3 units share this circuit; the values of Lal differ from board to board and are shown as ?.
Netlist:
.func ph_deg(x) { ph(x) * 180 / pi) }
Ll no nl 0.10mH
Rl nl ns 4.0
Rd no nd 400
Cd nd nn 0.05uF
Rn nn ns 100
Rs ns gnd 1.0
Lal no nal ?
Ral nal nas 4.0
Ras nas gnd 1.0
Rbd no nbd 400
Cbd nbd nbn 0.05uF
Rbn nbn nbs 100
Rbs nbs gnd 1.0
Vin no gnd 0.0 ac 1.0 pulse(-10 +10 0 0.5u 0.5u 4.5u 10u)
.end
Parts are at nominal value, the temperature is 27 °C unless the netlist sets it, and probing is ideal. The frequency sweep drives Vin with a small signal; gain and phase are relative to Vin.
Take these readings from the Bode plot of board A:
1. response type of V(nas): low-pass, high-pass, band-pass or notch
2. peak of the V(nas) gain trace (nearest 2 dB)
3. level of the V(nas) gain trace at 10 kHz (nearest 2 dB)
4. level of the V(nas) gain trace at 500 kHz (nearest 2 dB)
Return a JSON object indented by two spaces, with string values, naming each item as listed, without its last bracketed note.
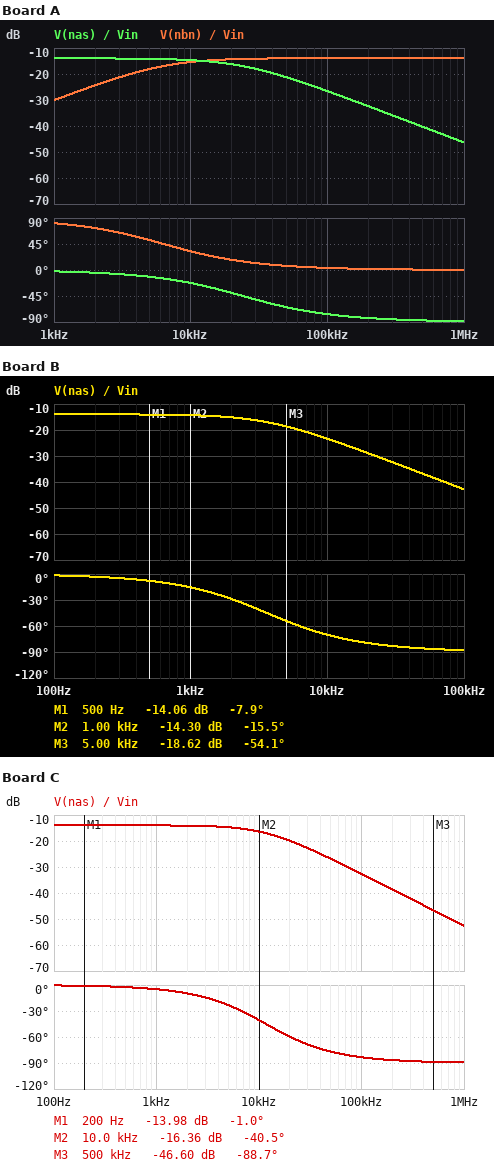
{
  "response type of V(nas): low-pass, high-pass, band-pass or notch": "low-pass",
  "peak of the V(nas) gain trace": "-14 dB",
  "level of the V(nas) gain trace at 10 kHz": "-14 dB",
  "level of the V(nas) gain trace at 500 kHz": "-40 dB"
}
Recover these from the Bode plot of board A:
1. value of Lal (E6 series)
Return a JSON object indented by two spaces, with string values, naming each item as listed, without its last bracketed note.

{
  "value of Lal": "33 µH"
}
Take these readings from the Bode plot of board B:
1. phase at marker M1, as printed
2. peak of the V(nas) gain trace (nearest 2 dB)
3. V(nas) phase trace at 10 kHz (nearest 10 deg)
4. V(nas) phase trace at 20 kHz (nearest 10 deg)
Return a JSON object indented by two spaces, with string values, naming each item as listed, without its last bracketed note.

{
  "phase at marker M1, as printed": "-7.9 deg",
  "peak of the V(nas) gain trace": "-14 dB",
  "V(nas) phase trace at 10 kHz": "-70 deg",
  "V(nas) phase trace at 20 kHz": "-80 deg"
}
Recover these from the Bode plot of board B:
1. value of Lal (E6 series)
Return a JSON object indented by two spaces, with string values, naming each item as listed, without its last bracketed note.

{
  "value of Lal": "220 µH"
}
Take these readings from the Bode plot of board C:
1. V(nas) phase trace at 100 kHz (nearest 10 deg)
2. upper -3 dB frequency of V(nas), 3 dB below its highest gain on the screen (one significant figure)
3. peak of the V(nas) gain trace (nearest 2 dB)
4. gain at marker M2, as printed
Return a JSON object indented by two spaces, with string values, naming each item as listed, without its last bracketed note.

{
  "V(nas) phase trace at 100 kHz": "-80 deg",
  "upper -3 dB frequency of V(nas), 3 dB below its highest gain on the screen": "10 kHz",
  "peak of the V(nas) gain trace": "-14 dB",
  "gain at marker M2, as printed": "-16.36 dB"
}
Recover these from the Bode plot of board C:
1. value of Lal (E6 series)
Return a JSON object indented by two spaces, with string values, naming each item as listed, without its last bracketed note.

{
  "value of Lal": "68 µH"
}
